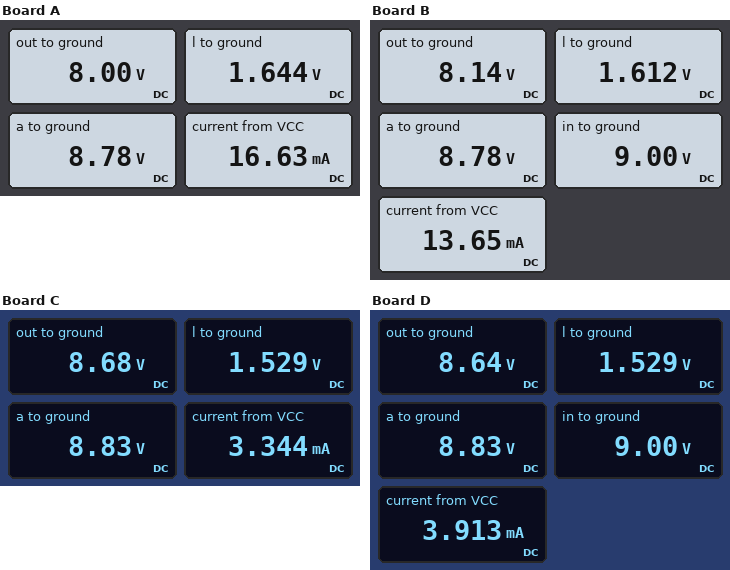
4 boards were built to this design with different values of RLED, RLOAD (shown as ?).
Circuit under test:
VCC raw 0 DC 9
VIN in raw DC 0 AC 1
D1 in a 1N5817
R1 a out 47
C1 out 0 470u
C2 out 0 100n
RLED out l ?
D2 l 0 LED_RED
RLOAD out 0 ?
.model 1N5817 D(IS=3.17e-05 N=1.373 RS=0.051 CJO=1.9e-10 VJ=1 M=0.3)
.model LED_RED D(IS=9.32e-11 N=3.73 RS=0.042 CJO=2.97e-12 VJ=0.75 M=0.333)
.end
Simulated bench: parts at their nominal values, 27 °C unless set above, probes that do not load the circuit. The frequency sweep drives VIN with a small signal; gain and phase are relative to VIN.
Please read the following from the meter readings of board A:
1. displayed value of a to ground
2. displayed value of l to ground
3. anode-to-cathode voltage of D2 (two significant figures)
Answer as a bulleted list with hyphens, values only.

- 8.78 V
- 1.644 V
- 1.6 V
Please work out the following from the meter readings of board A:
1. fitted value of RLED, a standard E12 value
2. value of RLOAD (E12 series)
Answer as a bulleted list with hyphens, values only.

- 2.7 kΩ
- 560 Ω
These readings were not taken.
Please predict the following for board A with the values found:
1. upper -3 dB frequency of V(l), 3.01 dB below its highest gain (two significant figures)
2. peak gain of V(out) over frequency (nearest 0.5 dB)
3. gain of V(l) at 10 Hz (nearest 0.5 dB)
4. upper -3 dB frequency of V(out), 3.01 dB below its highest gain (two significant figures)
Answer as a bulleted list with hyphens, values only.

- 7.6 Hz
- -1.0 dB
- -41.5 dB
- 7.6 Hz
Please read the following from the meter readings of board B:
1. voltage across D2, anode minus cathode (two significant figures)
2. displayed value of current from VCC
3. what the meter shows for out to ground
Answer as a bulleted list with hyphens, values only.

- 1.6 V
- 13.65 mA
- 8.14 V
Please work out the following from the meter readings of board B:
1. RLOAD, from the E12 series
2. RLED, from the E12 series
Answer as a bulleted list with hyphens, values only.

- 680 Ω
- 3.9 kΩ
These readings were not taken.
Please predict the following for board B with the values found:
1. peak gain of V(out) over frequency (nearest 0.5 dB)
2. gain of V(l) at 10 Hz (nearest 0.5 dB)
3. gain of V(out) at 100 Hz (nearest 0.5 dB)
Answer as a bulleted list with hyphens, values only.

- -0.5 dB
- -42.0 dB
- -23.5 dB
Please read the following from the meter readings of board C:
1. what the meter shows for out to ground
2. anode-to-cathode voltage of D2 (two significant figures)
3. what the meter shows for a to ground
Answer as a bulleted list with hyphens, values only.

- 8.68 V
- 1.5 V
- 8.83 V
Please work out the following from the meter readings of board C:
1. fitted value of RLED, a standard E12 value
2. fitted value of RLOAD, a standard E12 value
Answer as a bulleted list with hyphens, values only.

- 10 kΩ
- 3.3 kΩ
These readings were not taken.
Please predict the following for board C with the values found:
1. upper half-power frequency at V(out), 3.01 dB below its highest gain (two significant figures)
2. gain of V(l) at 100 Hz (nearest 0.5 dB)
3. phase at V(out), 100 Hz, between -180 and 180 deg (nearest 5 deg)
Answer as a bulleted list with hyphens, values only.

- 6.0 Hz
- -62.0 dB
- -85 deg
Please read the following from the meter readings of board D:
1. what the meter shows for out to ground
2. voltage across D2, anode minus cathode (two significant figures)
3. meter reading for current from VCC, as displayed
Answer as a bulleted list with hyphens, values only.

- 8.64 V
- 1.5 V
- 3.913 mA
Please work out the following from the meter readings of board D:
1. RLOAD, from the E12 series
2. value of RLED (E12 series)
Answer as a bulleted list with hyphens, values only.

- 2.7 kΩ
- 10 kΩ
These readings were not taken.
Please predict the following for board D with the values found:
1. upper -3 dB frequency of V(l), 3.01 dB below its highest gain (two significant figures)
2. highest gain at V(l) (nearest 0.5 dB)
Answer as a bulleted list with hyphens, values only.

- 6.2 Hz
- -37.5 dB
